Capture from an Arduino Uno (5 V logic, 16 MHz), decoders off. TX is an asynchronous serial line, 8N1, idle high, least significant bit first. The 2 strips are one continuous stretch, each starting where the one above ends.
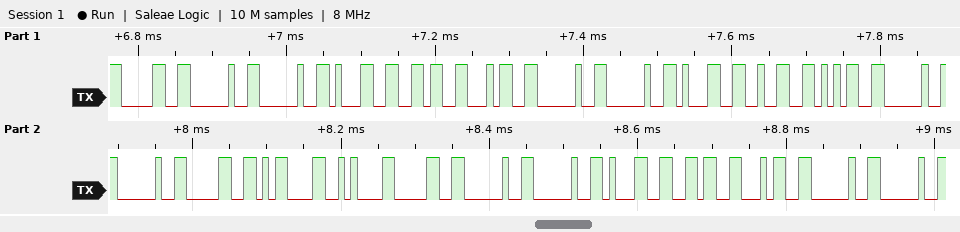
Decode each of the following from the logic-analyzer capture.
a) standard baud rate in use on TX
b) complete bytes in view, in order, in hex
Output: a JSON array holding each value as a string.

["115200 baud", "30 20 20 31 36 34 20 20 31 32 35 20 20 30 0D 0A 30 20 20 31 36 34 20 20"]
